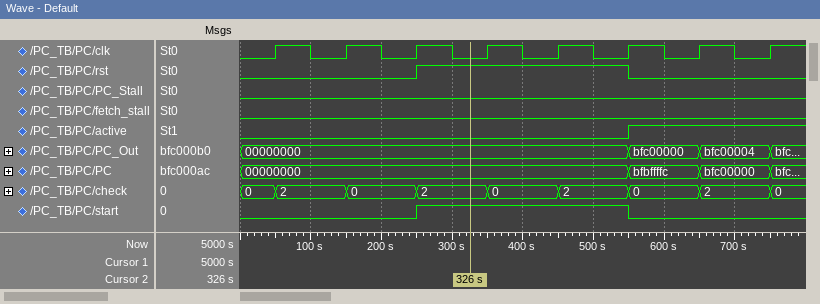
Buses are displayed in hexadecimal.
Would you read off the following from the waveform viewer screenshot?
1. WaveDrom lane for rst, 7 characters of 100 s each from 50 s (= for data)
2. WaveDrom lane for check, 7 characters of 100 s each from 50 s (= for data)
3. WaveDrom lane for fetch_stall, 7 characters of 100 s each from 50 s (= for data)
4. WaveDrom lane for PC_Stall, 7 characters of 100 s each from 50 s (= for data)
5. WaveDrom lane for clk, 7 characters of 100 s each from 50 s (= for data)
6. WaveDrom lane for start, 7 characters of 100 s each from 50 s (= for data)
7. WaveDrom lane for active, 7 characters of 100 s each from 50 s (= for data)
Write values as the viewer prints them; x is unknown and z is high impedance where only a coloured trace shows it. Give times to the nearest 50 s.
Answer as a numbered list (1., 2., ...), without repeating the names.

1. {name: 'rst', wave: '0.1..0.'}
2. {name: 'check', wave: '=======', data: '2 0 2 0 2 0 2'}
3. {name: 'fetch_stall', wave: '0......'}
4. {name: 'PC_Stall', wave: '0......'}
5. {name: 'clk', wave: 'p......'}
6. {name: 'start', wave: '0.1..0.'}
7. {name: 'active', wave: '0....1.'}
